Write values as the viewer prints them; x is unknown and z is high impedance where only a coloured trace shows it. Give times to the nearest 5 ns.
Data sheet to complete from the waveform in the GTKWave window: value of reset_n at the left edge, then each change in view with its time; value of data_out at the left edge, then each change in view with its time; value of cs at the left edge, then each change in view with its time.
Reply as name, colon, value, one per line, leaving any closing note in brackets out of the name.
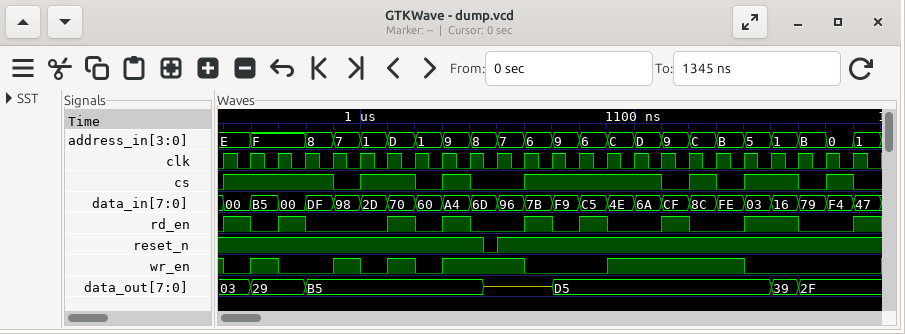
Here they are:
value of reset_n at the left edge, then each change in view with its time: 1, 0 at 1045 ns, 1 at 1050 ns
value of data_out at the left edge, then each change in view with its time: 03, 29 at 960 ns, B5 at 980 ns, z at 1045 ns, D5 at 1070 ns, 39 at 1150 ns, 2F at 1160 ns
value of cs at the left edge, then each change in view with its time: 0, 1 at 950 ns, 0 at 990 ns, 1 at 1000 ns, 0 at 1020 ns, 1 at 1030 ns, 0 at 1040 ns, 1 at 1060 ns, 0 at 1110 ns, 1 at 1120 ns, 0 at 1130 ns, 1 at 1140 ns, 0 at 1160 ns, 1 at 1170 ns, 0 at 1180 ns
